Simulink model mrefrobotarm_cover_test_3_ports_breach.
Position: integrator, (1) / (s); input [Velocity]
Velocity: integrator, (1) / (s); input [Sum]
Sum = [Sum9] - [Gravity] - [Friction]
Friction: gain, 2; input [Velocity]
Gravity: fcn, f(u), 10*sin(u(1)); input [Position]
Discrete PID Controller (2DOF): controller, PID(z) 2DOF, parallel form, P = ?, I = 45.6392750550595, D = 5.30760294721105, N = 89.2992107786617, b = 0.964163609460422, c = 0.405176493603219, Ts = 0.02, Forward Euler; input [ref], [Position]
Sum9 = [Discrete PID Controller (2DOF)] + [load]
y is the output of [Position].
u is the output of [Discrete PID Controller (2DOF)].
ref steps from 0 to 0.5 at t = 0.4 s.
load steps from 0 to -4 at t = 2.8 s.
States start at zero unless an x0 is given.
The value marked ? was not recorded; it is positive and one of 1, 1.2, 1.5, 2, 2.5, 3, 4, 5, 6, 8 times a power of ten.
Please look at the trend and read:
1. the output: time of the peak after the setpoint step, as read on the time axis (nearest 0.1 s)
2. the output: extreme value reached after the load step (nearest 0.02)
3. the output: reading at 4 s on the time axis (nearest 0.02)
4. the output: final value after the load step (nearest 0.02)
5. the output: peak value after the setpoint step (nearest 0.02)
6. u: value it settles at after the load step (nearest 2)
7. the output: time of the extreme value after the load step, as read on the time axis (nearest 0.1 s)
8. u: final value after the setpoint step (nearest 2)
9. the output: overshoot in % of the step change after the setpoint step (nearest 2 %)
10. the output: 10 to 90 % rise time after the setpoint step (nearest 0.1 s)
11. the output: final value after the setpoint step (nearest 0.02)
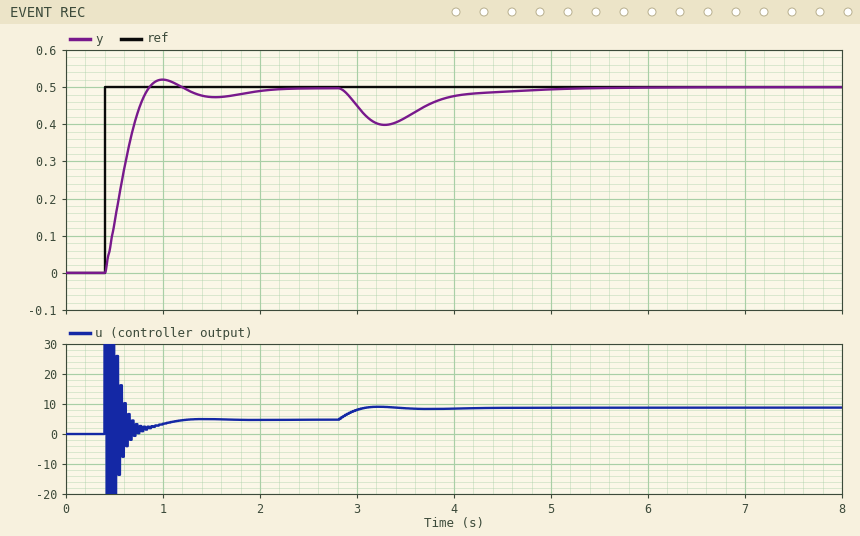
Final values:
1.0 s
0.40
0.48
0.50
0.52
8
3.3 s
4
4 %
0.3 s
0.50
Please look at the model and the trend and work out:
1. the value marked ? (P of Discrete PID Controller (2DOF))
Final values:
30
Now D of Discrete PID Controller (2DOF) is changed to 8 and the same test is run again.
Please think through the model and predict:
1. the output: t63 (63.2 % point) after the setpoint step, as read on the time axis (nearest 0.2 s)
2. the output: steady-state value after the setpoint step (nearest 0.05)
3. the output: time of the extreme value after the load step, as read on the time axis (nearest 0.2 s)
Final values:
0.6 s
0.50
3.4 s
